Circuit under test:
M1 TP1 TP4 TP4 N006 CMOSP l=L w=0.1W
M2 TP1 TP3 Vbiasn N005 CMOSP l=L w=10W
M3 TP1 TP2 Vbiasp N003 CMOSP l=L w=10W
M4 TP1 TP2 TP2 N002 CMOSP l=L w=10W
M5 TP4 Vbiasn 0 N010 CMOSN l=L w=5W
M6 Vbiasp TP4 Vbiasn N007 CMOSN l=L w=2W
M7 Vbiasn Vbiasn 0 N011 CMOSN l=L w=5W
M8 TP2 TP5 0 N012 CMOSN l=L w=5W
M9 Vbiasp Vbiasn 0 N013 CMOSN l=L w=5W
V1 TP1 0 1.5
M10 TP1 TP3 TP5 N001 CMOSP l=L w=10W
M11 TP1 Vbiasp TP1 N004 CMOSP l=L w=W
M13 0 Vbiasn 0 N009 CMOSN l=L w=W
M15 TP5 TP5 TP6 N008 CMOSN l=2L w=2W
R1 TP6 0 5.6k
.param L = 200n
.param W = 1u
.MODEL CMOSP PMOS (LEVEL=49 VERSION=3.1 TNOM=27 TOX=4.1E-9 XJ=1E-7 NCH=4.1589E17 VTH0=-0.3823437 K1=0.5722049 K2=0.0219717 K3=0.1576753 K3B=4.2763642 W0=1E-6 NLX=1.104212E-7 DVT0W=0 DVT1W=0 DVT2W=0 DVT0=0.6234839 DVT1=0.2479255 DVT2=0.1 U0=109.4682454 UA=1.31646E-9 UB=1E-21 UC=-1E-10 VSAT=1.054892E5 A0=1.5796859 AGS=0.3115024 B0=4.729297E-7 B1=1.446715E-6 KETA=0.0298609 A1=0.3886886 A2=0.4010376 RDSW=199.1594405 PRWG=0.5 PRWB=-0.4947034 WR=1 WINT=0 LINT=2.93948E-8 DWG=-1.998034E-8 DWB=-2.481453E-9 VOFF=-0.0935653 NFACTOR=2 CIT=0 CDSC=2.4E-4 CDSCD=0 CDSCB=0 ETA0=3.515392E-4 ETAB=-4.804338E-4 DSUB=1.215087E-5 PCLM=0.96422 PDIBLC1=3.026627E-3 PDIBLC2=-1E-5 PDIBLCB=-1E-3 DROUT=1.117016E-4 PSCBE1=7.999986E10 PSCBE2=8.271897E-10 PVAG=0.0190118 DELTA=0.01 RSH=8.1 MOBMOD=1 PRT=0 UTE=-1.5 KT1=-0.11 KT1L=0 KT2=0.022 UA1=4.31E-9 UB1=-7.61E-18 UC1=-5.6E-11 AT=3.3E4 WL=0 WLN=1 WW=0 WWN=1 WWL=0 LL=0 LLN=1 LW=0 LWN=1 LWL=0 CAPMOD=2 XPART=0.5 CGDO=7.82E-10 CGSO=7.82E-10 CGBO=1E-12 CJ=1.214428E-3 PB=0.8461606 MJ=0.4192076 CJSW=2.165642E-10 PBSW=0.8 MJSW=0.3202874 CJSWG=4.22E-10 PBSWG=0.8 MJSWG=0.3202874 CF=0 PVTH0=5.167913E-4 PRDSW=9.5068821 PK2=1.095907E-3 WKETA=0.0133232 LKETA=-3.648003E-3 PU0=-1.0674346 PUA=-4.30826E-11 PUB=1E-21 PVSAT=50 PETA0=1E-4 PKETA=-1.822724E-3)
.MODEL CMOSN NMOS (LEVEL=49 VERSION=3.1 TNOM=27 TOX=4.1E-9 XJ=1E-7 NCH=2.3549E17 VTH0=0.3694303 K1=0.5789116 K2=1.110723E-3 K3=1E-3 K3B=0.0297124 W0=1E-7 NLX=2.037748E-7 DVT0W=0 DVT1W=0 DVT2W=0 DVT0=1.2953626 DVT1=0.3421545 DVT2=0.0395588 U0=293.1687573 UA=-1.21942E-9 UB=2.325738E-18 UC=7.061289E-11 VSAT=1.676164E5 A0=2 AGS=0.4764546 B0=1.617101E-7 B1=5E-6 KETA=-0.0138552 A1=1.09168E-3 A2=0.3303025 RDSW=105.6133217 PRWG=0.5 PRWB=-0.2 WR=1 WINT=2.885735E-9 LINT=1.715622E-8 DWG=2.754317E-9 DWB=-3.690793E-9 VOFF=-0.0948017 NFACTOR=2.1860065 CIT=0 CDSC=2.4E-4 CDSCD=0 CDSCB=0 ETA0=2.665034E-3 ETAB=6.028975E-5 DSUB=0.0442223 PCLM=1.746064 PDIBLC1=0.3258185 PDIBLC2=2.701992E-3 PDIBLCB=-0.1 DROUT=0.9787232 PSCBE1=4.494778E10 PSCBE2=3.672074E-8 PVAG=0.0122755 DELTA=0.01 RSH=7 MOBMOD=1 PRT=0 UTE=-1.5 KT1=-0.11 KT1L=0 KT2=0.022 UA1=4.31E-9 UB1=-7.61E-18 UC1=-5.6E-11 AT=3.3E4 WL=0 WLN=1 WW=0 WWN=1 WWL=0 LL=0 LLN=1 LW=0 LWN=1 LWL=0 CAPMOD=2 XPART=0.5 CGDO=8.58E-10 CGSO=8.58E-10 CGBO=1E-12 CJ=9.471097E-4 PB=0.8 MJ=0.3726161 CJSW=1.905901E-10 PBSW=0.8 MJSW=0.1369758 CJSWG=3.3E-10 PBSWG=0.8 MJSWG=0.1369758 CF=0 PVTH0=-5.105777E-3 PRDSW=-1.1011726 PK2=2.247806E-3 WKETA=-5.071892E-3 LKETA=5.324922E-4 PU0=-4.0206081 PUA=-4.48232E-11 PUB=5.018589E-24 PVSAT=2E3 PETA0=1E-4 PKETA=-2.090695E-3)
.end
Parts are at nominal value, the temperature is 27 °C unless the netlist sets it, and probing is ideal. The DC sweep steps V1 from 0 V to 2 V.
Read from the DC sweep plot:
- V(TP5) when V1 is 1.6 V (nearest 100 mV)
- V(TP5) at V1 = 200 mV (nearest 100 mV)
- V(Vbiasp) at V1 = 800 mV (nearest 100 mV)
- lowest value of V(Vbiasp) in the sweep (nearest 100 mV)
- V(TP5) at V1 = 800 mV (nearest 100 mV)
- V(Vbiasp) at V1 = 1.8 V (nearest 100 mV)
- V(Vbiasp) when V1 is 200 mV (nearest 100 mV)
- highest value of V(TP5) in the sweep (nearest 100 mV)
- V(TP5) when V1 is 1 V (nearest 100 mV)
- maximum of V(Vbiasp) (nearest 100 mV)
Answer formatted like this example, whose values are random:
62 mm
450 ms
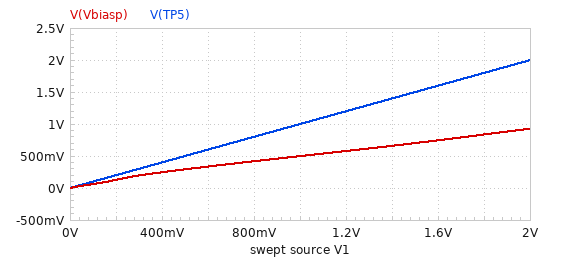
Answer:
1.6 V
200 mV
400 mV
0 V
800 mV
800 mV
100 mV
2.0 V
1.0 V
900 mV
